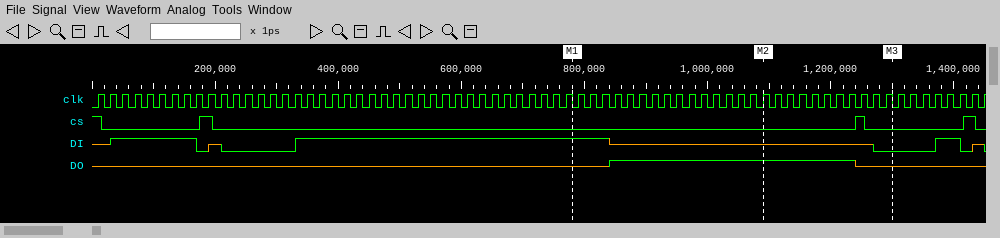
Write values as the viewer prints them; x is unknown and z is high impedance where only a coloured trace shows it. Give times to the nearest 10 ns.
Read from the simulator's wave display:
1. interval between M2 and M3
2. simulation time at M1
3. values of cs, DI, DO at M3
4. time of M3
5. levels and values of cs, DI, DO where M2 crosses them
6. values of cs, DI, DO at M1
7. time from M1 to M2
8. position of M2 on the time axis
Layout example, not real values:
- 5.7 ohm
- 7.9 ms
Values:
- 210 ns
- 780 ns
- cs=0, DI=0, DO=z
- 1300 ns
- cs=0, DI=z, DO=1
- cs=0, DI=1, DO=z
- 310 ns
- 1090 ns
